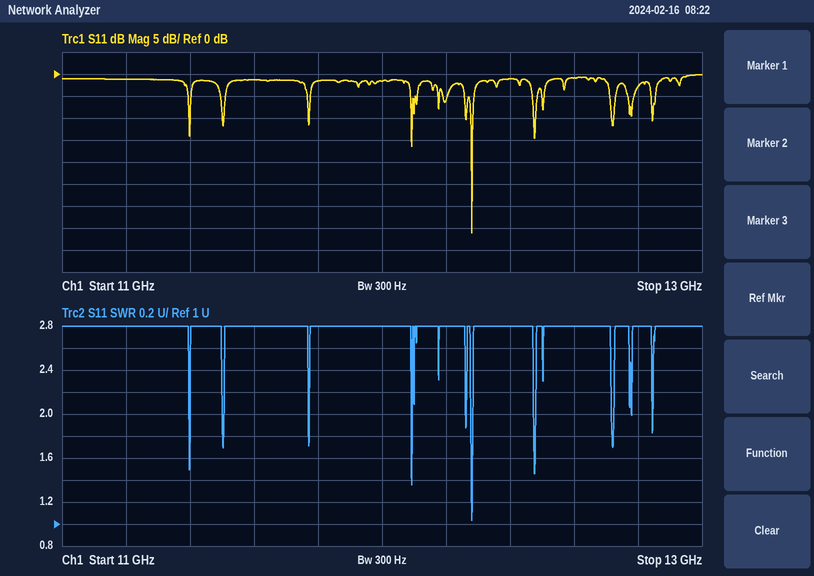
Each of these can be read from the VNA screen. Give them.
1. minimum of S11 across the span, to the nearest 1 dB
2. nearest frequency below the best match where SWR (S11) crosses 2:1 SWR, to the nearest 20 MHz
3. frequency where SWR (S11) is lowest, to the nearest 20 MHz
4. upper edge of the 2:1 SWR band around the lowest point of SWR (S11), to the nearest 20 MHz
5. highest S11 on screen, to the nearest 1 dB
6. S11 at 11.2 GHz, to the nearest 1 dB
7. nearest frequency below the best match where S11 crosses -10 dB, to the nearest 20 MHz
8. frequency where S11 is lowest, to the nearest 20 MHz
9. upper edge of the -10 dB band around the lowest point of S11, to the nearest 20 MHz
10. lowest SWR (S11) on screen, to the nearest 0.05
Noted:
-36 dB
12.28 GHz
12.28 GHz
12.28 GHz
0 dB
-1 dB
12.28 GHz
12.28 GHz
12.28 GHz
1.05
